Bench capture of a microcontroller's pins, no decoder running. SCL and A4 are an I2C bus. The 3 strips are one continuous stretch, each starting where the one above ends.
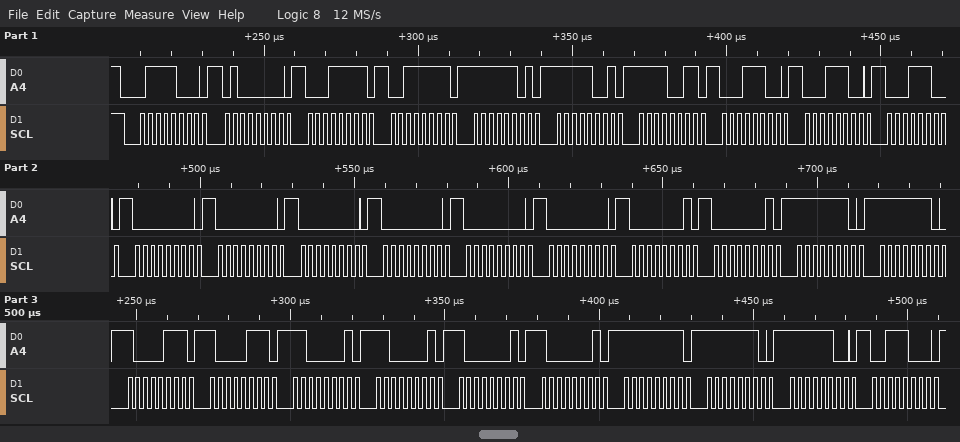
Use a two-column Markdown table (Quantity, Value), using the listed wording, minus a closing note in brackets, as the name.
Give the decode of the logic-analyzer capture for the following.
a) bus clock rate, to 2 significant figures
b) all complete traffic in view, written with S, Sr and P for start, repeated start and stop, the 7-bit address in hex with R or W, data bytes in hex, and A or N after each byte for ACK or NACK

| Quantity | Value |
|---|---|
| bus clock rate, to 2 significant figures | 400 kHz |
| all complete traffic in view, written with S, Sr and P for start, repeated start and stop, the 7-bit address in hex with R or W, data bytes in hex, and A or N after each byte for ACK or NACK | S 3CW A 40 A 1F A 3F A FD A F9 A F3 A 1C A 1C A 1C A 00 A 00 A 00 A 00 A 00 A 00 A 01 A 01 A FE A FE A 87 A 87 A C1 A C1 A 81 A 81 A FF A FE A FC A 38 A |
